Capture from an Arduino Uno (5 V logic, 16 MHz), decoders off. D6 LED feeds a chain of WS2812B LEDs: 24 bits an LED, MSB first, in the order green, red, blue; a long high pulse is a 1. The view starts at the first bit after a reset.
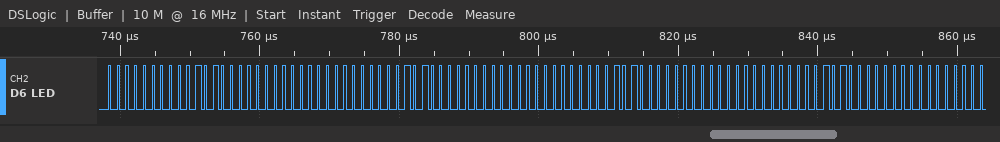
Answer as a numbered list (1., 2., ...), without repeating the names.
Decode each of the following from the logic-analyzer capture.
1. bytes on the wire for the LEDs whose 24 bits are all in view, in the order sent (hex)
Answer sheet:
1. 00 28 00 00 28 00 00 28 00 00 28 00
